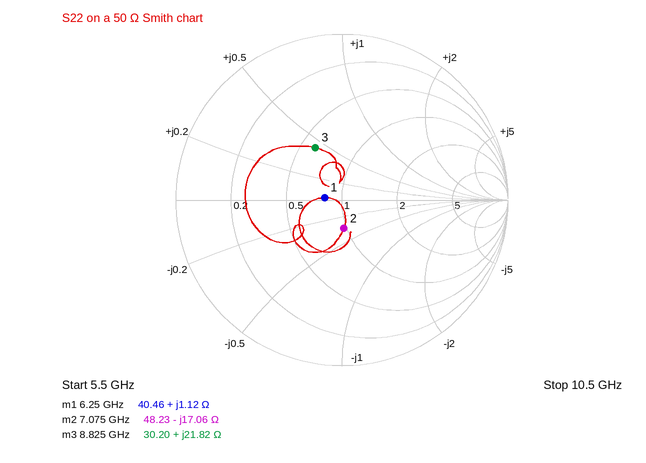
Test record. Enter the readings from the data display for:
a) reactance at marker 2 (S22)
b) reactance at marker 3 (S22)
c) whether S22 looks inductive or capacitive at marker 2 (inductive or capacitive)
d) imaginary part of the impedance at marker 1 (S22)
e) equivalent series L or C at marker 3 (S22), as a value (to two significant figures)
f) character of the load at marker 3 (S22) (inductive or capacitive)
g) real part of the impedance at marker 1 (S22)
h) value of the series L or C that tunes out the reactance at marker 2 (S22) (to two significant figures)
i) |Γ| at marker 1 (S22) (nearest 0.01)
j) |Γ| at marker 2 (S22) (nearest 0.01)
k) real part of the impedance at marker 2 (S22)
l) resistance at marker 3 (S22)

-17.06 Ω
+21.82 Ω
capacitive
+1.12 Ω
390 pH
inductive
40.46 Ω
380 pH
0.11
0.17
48.23 Ω
30.20 Ω
